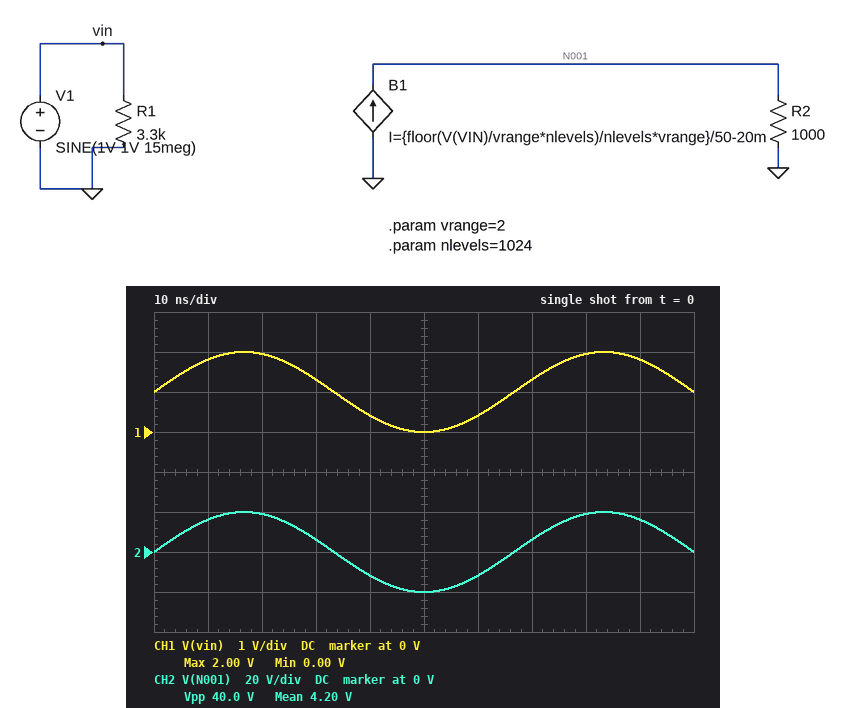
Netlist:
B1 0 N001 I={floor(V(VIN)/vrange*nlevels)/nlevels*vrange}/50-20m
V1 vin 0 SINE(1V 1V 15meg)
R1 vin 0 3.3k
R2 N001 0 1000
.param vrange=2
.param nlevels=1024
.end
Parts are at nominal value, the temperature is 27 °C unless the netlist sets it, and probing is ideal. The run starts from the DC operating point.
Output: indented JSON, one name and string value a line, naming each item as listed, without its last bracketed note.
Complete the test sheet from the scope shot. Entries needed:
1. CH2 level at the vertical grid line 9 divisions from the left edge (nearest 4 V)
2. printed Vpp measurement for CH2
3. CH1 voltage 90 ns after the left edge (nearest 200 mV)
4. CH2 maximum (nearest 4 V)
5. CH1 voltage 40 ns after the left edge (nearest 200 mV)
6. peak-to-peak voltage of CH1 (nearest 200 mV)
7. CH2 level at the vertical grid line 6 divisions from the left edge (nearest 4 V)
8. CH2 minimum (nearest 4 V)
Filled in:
{
  "CH2 level at the vertical grid line 9 divisions from the left edge": "16 V",
  "printed Vpp measurement for CH2": "40.0 V",
  "CH1 voltage 90 ns after the left edge": "1.8 V",
  "CH2 maximum": "20 V",
  "CH1 voltage 40 ns after the left edge": "400 mV",
  "peak-to-peak voltage of CH1": "2.0 V",
  "CH2 level at the vertical grid line 6 divisions from the left edge": "-12 V",
  "CH2 minimum": "-20 V"
}
